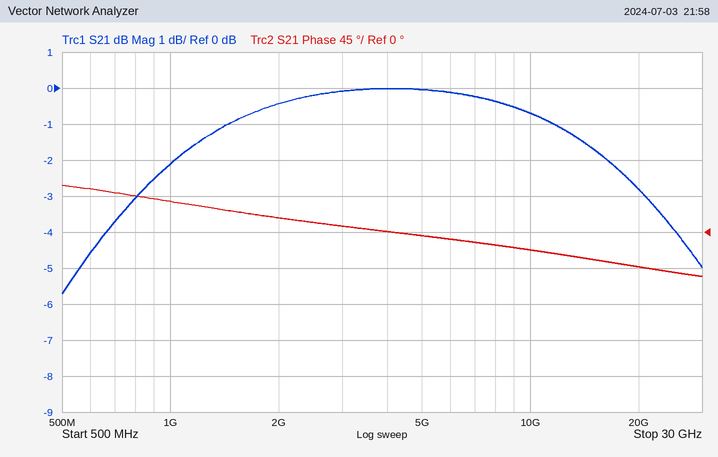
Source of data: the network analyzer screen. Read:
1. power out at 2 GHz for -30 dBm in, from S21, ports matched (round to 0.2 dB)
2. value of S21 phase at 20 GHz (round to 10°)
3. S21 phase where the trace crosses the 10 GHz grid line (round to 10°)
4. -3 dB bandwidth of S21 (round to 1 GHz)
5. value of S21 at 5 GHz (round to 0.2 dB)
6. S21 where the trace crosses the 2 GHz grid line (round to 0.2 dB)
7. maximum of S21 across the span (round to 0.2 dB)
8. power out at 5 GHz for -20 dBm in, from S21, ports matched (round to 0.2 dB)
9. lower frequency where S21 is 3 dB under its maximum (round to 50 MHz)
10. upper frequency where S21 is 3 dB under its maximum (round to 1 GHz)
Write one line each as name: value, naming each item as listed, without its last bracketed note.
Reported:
power out at 2 GHz for -30 dBm in, from S21, ports matched: -30.4 dBm
value of S21 phase at 20 GHz: -40°
S21 phase where the trace crosses the 10 GHz grid line: -20°
-3 dB bandwidth of S21: 20 GHz
value of S21 at 5 GHz: 0.0 dB
S21 where the trace crosses the 2 GHz grid line: -0.4 dB
maximum of S21 across the span: 0.0 dB
power out at 5 GHz for -20 dBm in, from S21, ports matched: -20.0 dBm
lower frequency where S21 is 3 dB under its maximum: 800 MHz
upper frequency where S21 is 3 dB under its maximum: 21 GHz
